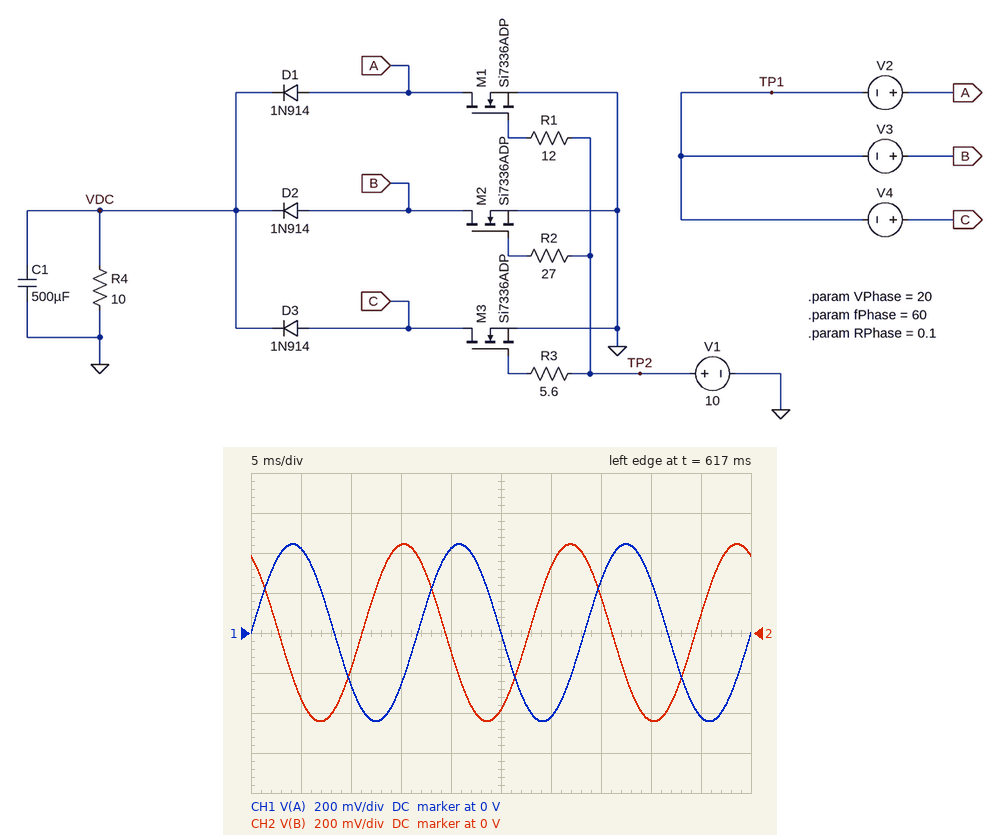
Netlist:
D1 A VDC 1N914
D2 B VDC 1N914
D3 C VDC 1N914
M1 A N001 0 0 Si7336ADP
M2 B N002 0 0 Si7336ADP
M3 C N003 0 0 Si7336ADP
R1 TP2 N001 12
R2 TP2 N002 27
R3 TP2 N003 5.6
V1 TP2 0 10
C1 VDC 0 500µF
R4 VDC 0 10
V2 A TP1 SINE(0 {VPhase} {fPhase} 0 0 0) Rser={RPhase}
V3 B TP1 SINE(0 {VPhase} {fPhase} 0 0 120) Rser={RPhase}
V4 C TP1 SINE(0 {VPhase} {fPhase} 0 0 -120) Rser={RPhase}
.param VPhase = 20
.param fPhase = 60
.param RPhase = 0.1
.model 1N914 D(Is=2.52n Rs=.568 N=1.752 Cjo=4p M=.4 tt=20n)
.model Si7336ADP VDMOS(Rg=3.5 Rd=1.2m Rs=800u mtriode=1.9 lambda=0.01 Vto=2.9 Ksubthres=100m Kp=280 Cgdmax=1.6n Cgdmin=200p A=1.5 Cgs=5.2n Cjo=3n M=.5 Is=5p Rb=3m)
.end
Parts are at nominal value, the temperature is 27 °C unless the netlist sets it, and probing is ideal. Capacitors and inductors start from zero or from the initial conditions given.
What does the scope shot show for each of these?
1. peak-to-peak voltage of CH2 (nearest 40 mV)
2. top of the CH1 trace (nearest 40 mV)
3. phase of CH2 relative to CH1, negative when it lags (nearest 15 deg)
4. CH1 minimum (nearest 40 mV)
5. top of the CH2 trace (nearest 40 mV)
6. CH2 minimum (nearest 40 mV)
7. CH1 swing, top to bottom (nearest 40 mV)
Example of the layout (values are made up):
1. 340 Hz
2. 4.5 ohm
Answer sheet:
1. 880 mV
2. 440 mV
3. 120 deg
4. -440 mV
5. 440 mV
6. -440 mV
7. 880 mV
